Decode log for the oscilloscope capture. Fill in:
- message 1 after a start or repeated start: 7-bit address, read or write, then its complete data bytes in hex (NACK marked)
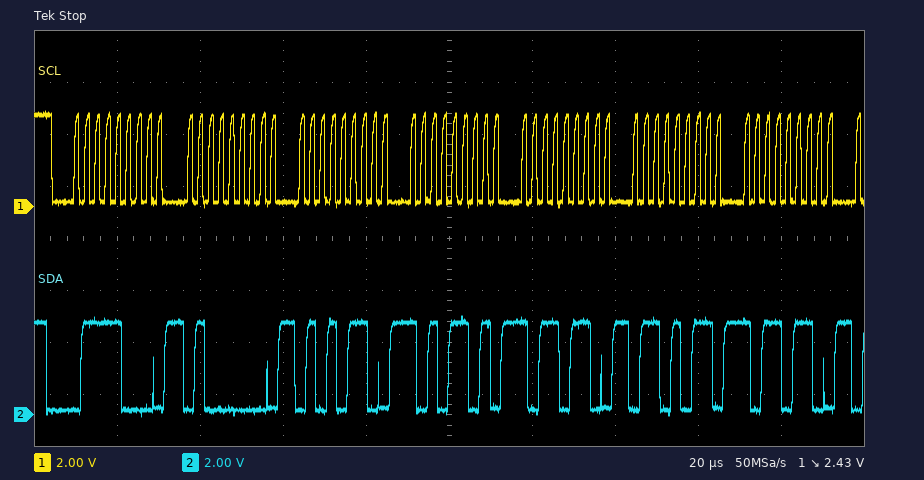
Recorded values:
0x3C write: 40 56 AD B6 6B B6
